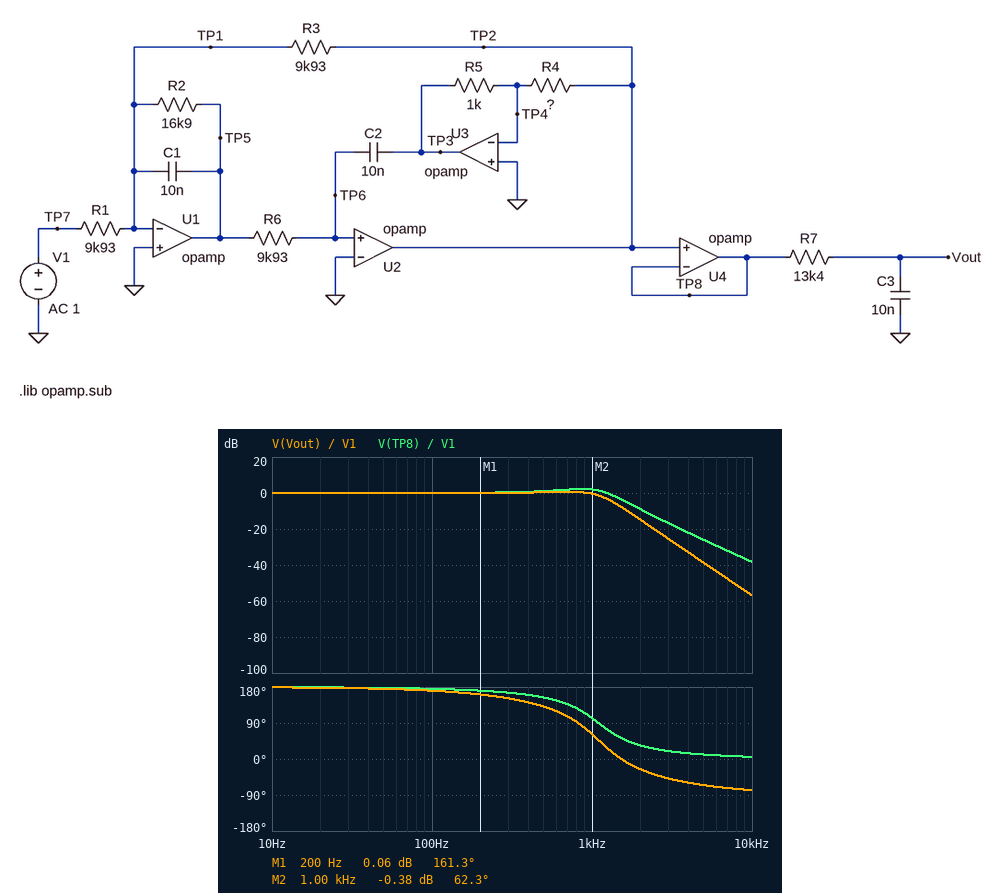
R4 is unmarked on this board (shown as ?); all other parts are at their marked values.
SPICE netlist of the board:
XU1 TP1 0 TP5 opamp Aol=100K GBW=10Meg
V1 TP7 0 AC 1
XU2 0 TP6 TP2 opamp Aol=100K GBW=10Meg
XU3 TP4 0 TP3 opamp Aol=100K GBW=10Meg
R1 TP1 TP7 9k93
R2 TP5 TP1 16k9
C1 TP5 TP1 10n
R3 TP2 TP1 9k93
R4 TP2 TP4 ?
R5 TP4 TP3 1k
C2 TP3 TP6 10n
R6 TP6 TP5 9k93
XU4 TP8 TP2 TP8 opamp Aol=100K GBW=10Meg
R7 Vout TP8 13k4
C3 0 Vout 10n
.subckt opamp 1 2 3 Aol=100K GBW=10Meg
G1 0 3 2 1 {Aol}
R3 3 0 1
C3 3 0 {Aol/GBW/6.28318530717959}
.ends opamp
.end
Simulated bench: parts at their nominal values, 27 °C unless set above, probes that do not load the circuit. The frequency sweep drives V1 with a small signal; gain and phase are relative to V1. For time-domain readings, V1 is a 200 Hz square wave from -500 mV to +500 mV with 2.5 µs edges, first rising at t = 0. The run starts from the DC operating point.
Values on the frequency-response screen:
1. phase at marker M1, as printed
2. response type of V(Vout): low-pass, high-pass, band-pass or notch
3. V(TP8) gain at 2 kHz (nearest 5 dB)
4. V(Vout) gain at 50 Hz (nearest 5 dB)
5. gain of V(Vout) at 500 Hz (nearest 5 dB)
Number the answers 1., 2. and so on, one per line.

1. 161.3 deg
2. low-pass
3. -10 dB
4. 0 dB
5. 0 dB
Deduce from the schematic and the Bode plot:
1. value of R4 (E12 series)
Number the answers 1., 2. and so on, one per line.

1. 470 Ω
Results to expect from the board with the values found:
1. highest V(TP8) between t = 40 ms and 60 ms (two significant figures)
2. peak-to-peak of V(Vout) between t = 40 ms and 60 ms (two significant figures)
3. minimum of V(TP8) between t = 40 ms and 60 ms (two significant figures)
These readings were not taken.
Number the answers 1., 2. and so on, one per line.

1. 730 mV
2. 1.3 V
3. -730 mV
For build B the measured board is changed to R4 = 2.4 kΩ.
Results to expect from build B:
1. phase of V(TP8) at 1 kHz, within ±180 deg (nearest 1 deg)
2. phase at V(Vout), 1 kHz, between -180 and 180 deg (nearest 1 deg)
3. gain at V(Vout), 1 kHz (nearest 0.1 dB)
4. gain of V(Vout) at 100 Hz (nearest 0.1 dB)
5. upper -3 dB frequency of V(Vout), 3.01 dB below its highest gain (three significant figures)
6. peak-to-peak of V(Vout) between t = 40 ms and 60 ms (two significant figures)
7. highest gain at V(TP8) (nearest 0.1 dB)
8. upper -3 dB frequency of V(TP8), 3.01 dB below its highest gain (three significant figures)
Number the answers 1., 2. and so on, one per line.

1. 170 deg
2. 130 deg
3. -0.9 dB
4. 0 dB
5. 2.73 kHz
6. 1.2 V
7. 8.6 dB
8. 2.83 kHz
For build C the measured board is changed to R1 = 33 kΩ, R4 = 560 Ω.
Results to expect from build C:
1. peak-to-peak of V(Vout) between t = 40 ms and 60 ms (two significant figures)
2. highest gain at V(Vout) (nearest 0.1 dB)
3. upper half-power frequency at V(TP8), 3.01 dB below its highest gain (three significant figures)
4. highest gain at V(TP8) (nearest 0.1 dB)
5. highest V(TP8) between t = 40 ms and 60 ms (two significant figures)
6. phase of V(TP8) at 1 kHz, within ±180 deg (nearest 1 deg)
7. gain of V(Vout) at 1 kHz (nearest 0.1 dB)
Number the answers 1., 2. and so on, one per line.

1. 390 mV
2. -9.7 dB
3. 1.43 kHz
4. -7.6 dB
5. 230 mV
6. 115 deg
7. -9.9 dB
